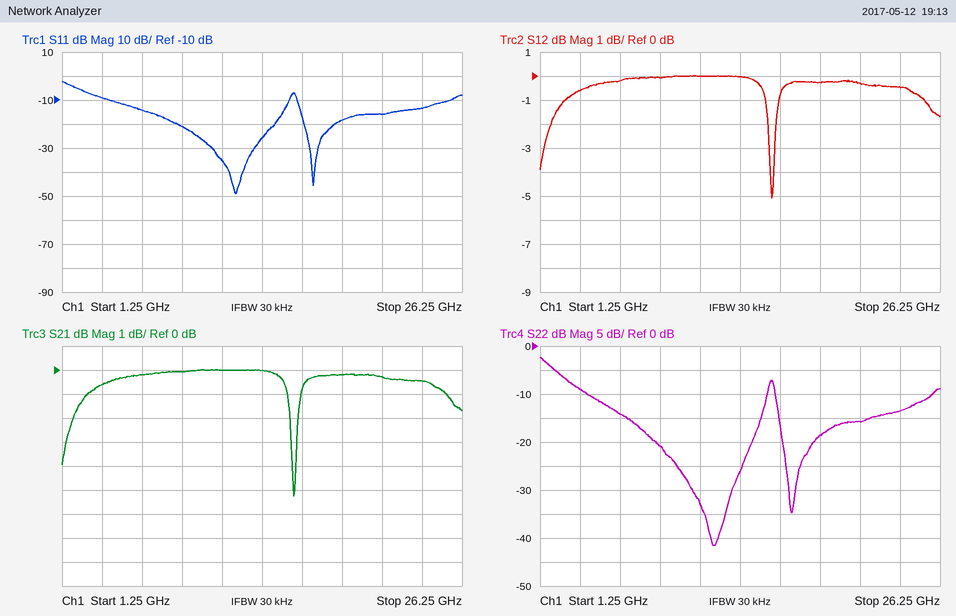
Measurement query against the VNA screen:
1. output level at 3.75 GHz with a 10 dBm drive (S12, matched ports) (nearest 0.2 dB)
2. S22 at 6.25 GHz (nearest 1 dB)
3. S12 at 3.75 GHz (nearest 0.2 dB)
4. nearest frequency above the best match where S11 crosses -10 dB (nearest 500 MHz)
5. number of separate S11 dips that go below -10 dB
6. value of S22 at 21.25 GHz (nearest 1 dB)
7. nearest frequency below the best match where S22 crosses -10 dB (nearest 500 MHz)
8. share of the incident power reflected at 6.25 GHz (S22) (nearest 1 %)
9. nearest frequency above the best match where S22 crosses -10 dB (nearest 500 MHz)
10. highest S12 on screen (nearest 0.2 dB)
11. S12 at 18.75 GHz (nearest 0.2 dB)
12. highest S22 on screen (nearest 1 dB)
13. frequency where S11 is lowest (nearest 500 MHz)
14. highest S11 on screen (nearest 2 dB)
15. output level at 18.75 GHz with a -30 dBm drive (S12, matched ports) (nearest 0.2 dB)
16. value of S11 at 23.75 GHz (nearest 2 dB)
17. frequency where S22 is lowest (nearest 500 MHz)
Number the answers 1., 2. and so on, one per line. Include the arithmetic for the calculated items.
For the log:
1. 10 dBm + (-0.6 dB) = 9.4 dBm
2. -14 dB
3. -0.6 dB
4. 15.5 GHz
5. 2
6. -16 dB
7. 4.0 GHz
8. 10^(-14/10) ≈ 4 %
9. 15.5 GHz
10. 0.0 dB
11. -0.2 dB
12. -2 dB
13. 12.0 GHz
14. -2 dB
15. -30 dBm + (-0.2 dB) = -30.2 dBm
16. -14 dB
17. 12.0 GHz
